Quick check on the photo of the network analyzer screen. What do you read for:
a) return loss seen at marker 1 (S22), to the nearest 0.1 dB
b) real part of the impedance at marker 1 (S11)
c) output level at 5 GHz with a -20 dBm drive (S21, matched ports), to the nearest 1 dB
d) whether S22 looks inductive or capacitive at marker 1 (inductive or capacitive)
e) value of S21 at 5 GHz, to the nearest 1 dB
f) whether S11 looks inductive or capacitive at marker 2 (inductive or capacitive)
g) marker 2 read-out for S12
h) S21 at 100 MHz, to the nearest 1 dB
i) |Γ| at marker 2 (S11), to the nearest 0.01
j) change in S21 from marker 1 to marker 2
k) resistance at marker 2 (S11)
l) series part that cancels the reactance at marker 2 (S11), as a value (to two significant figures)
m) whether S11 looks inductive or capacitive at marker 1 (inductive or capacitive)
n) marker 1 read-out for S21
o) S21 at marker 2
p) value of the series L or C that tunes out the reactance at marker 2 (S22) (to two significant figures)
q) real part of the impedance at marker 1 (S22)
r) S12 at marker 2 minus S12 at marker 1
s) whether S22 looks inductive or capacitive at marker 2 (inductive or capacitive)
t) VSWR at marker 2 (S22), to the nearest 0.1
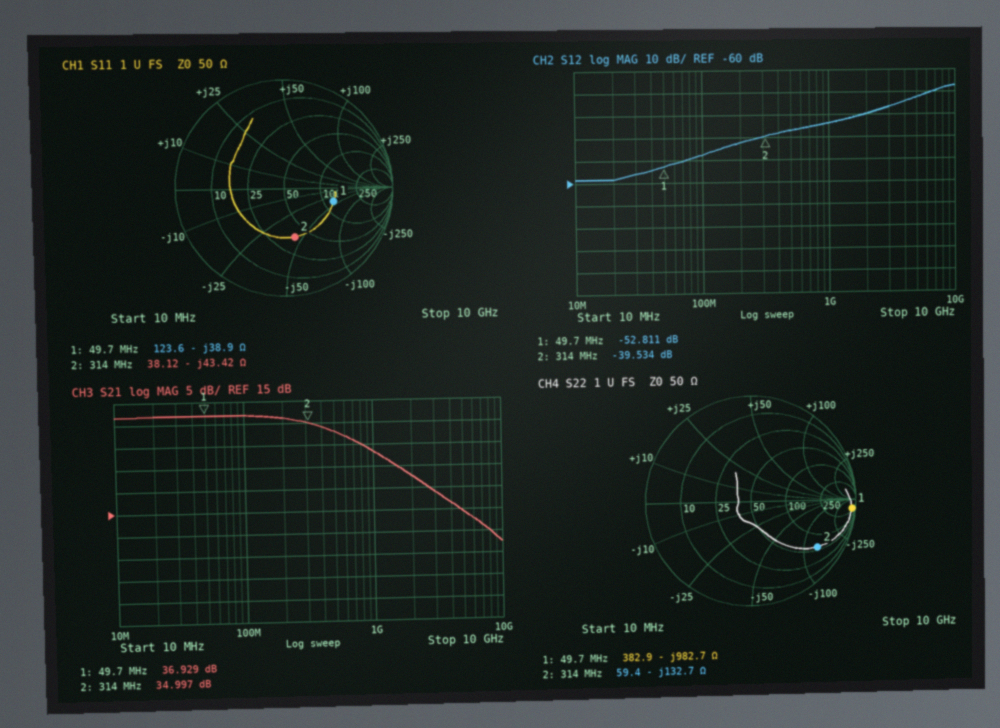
0.3 dB
123.6 Ω
-6 dBm
capacitive
14 dB
capacitive
-39.534 dB
37 dB
0.46
-1.932 dB
38.12 Ω
22 nH
capacitive
36.929 dB
34.997 dB
67 nH
382.9 Ω
13.277 dB
capacitive
7.8
